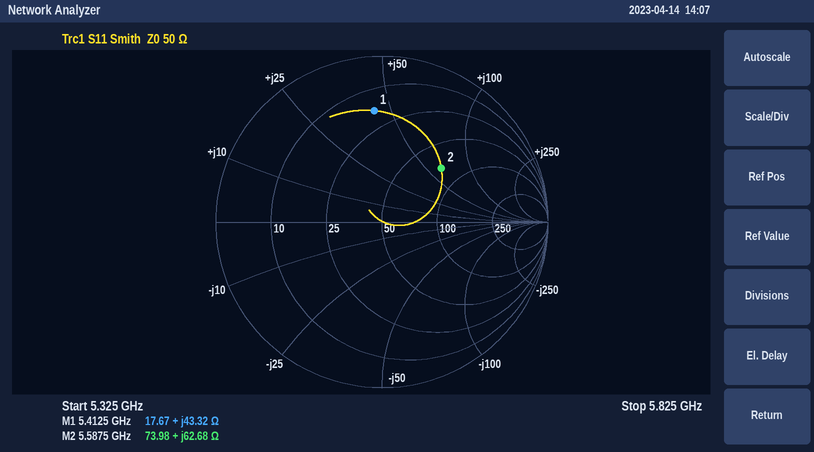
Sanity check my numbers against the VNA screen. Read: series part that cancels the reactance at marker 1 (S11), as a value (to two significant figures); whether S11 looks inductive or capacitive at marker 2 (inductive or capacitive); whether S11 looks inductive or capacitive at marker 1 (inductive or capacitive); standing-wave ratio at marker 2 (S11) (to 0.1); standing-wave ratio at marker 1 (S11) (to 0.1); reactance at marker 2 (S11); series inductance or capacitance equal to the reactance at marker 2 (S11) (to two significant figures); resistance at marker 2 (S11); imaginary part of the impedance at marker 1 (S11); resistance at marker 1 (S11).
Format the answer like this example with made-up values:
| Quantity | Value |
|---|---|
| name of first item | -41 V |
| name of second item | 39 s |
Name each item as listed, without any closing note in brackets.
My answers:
| Quantity | Value |
|---|---|
| series part that cancels the reactance at marker 1 (S11), as a value | 680 fF |
| whether S11 looks inductive or capacitive at marker 2 | inductive |
| whether S11 looks inductive or capacitive at marker 1 | inductive |
| standing-wave ratio at marker 2 (S11) | 2.9 |
| standing-wave ratio at marker 1 (S11) | 5.1 |
| reactance at marker 2 | +62.68 Ω |
| series inductance or capacitance equal to the reactance at marker 2 (S11) | 1.8 nH |
| resistance at marker 2 | 73.98 Ω |
| imaginary part of the impedance at marker 1 | +43.32 Ω |
| resistance at marker 1 | 17.67 Ω |
